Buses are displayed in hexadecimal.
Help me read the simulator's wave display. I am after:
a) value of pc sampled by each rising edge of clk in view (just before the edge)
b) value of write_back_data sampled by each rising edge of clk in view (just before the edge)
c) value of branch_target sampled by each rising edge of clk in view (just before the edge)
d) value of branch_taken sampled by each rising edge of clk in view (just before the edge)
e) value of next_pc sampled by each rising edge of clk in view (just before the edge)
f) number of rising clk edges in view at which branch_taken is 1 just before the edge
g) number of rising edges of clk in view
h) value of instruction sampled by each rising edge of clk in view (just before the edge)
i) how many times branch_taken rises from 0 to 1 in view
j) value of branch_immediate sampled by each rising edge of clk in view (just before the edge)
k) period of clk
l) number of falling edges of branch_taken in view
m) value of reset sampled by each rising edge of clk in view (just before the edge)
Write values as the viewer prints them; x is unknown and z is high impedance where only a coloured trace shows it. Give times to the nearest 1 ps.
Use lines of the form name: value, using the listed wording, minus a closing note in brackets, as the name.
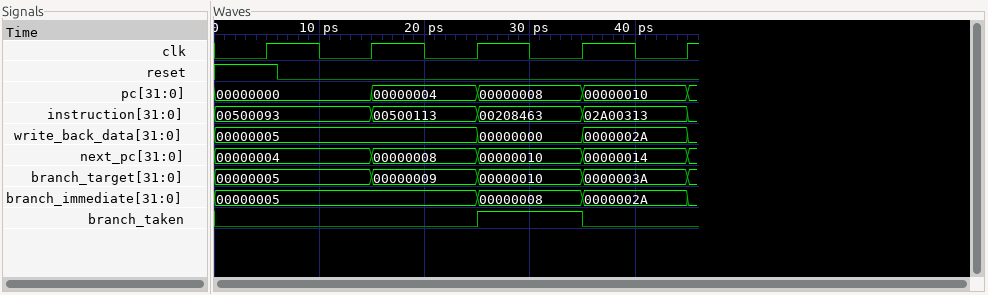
value of pc sampled by each rising edge of clk in view: 00000000, 00000000, 00000004, 00000008, 00000010
value of write_back_data sampled by each rising edge of clk in view: 00000005, 00000005, 00000005, 00000000, 0000002A
value of branch_target sampled by each rising edge of clk in view: 00000005, 00000005, 00000009, 00000010, 0000003A
value of branch_taken sampled by each rising edge of clk in view: 0 0 0 1 0
value of next_pc sampled by each rising edge of clk in view: 00000004, 00000004, 00000008, 00000010, 00000014
number of rising clk edges in view at which branch_taken is 1 just before the edge: 1
number of rising edges of clk in view: 5
value of instruction sampled by each rising edge of clk in view: 00500093, 00500093, 00500113, 00208463, 02A00313
how many times branch_taken rises from 0 to 1 in view: 1
value of branch_immediate sampled by each rising edge of clk in view: 00000005, 00000005, 00000005, 00000008, 0000002A
period of clk: 10 ps
number of falling edges of branch_taken in view: 1
value of reset sampled by each rising edge of clk in view: 1 0 0 0 0
